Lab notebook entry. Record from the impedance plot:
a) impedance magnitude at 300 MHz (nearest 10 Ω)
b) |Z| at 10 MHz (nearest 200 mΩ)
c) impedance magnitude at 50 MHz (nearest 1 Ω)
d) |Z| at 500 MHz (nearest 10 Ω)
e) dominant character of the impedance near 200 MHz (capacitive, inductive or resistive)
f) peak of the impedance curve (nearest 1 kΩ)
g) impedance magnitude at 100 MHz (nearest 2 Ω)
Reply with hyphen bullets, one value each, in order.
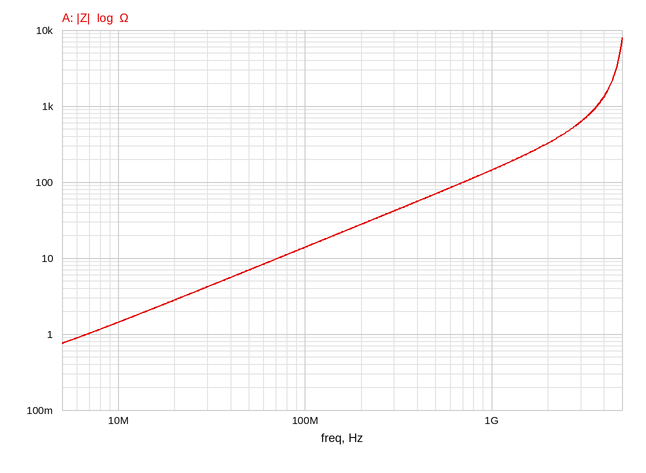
- 40 Ω
- 1.4 Ω
- 7 Ω
- 70 Ω
- inductive
- 8 kΩ
- 14 Ω
